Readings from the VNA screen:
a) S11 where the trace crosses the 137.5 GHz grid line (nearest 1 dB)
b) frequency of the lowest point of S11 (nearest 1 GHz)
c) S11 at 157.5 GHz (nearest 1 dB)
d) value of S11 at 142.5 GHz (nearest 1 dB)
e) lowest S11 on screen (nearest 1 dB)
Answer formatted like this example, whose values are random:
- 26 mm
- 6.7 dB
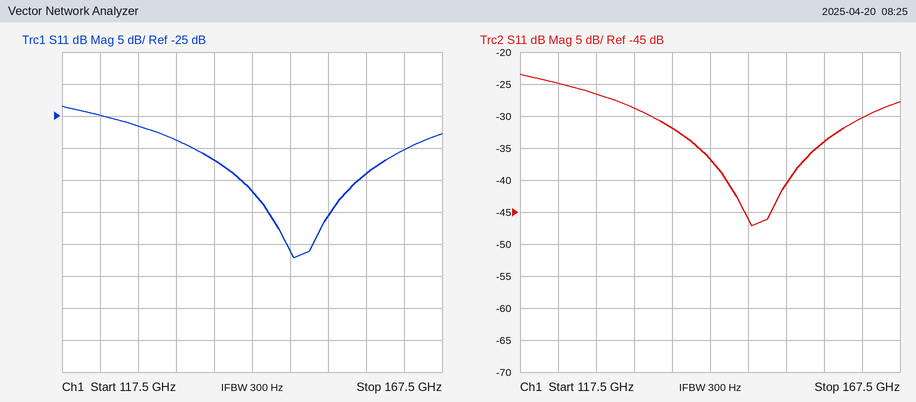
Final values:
- -32 dB
- 148 GHz
- -34 dB
- -37 dB
- -47 dB
